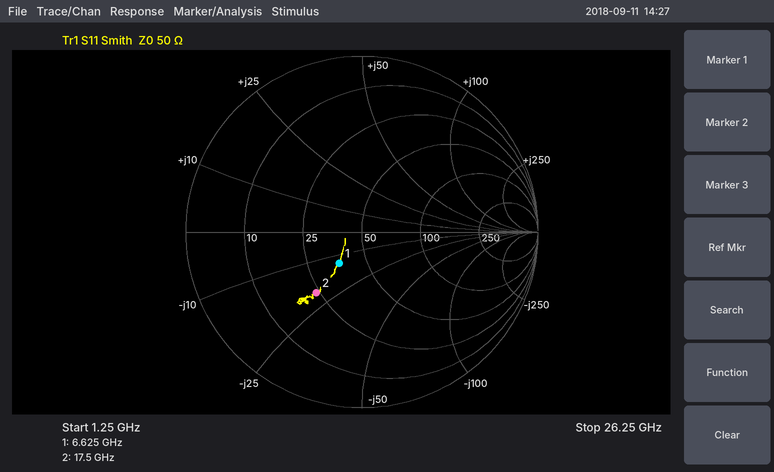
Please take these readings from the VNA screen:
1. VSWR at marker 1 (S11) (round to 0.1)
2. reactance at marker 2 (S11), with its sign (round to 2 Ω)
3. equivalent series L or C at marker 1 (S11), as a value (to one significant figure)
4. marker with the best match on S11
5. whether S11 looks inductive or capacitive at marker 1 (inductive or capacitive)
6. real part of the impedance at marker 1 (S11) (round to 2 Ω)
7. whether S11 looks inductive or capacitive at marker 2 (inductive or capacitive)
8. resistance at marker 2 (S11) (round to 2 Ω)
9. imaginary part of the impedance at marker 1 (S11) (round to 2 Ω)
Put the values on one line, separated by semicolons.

1.6; -20 Ω; 2 pF; marker 1; capacitive; 36 Ω; capacitive; 24 Ω; -14 Ω
